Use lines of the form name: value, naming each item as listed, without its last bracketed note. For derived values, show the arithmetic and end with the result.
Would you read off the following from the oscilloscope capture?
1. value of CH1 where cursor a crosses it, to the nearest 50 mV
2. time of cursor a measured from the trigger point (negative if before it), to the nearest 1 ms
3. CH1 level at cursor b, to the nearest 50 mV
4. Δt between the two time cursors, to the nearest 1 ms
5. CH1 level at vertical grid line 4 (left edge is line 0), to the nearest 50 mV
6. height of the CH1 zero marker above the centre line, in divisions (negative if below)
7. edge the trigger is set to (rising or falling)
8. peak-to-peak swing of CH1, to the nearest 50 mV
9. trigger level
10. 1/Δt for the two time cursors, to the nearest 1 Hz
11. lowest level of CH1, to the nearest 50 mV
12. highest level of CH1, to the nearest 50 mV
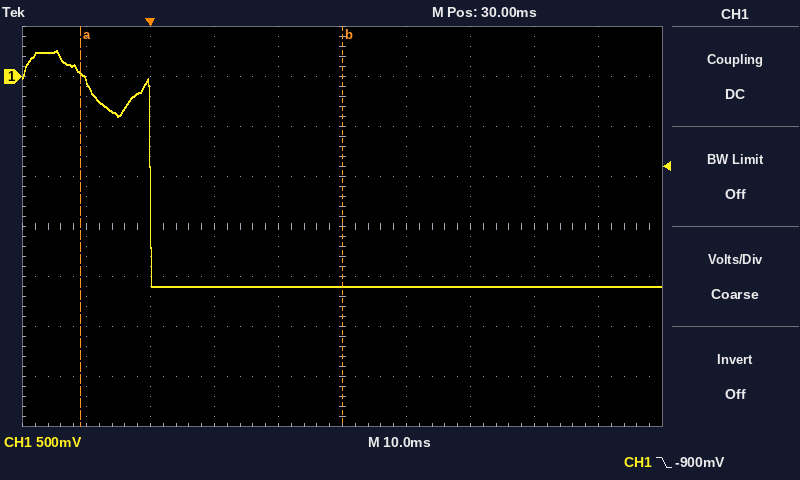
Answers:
value of CH1 where cursor a crosses it, to the nearest 50 mV: 50 mV
time of cursor a measured from the trigger point (negative if before it), to the nearest 1 ms: -11 ms
CH1 level at cursor b, to the nearest 50 mV: -2.10 V
Δt between the two time cursors, to the nearest 1 ms: 41 ms
CH1 level at vertical grid line 4 (left edge is line 0), to the nearest 50 mV: -2.10 V
height of the CH1 zero marker above the centre line, in divisions: +3.0 div
edge the trigger is set to: falling
peak-to-peak swing of CH1, to the nearest 50 mV: 250 mV − (-2.10 V) = 2.35 V
trigger level: -900 mV
1/Δt for the two time cursors, to the nearest 1 Hz: 1 / 41 ms ≈ 24 Hz
lowest level of CH1, to the nearest 50 mV: -2.10 V
highest level of CH1, to the nearest 50 mV: 250 mV
